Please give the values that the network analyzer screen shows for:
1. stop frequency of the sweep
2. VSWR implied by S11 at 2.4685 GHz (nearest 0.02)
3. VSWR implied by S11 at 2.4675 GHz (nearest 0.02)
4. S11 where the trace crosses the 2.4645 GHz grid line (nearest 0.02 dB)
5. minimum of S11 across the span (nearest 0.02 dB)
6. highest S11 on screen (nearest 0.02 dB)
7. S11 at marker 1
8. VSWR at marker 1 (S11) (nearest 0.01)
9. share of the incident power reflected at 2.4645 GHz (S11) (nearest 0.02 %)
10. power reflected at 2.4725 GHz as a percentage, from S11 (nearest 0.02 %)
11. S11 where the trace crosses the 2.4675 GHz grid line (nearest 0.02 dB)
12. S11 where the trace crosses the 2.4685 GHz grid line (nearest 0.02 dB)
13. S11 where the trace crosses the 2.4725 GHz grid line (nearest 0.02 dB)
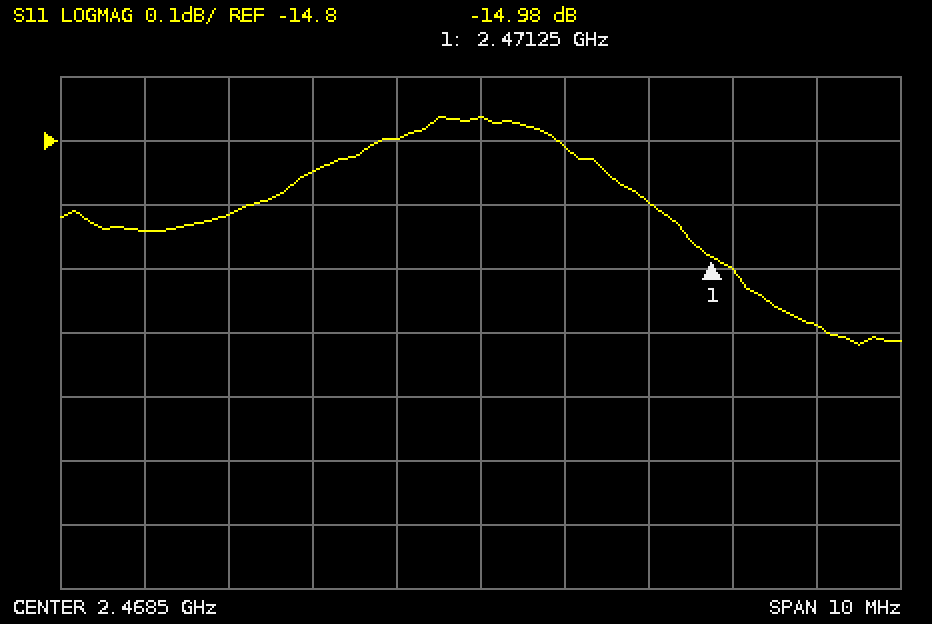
2.4735 GHz
1.44
1.44
-14.94 dB
-15.12 dB
-14.76 dB
-14.98 dB
1.43
3.20 %
3.10 %
-14.80 dB
-14.76 dB
-15.08 dB
